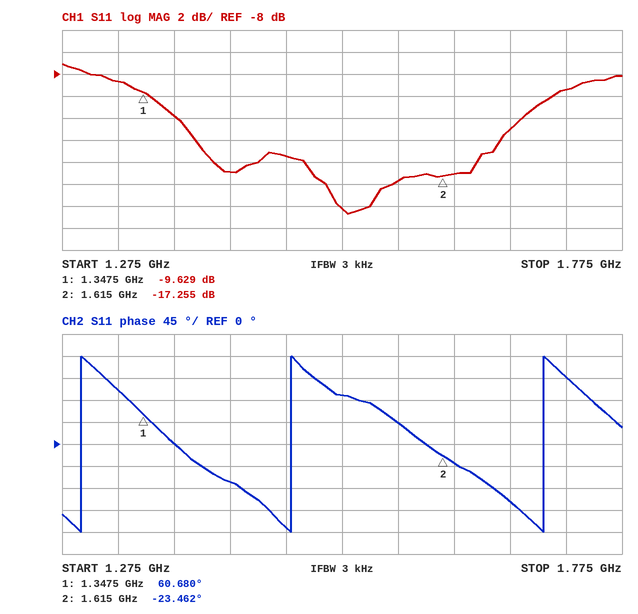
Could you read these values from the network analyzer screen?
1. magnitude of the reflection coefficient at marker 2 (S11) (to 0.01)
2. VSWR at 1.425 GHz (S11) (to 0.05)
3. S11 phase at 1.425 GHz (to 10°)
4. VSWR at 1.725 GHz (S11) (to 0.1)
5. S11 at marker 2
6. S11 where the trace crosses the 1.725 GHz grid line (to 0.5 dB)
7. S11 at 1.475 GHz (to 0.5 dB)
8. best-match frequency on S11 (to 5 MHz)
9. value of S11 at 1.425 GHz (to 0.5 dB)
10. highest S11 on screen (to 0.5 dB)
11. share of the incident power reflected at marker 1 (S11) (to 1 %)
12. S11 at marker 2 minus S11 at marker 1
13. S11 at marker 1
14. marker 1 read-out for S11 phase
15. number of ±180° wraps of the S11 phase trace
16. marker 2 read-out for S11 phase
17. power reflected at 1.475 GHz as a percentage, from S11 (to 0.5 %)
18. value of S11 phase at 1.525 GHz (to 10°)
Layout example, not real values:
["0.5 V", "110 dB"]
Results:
["0.14", "1.35", "-80°", "2.0", "-17.255 dB", "-9.5 dB", "-15.5 dB", "1.530 GHz", "-17.0 dB", "-7.0 dB", "11 %", "-7.626 dB", "-9.629 dB", "60.680°", "3", "-23.462°", "3.0 %", "100°"]
